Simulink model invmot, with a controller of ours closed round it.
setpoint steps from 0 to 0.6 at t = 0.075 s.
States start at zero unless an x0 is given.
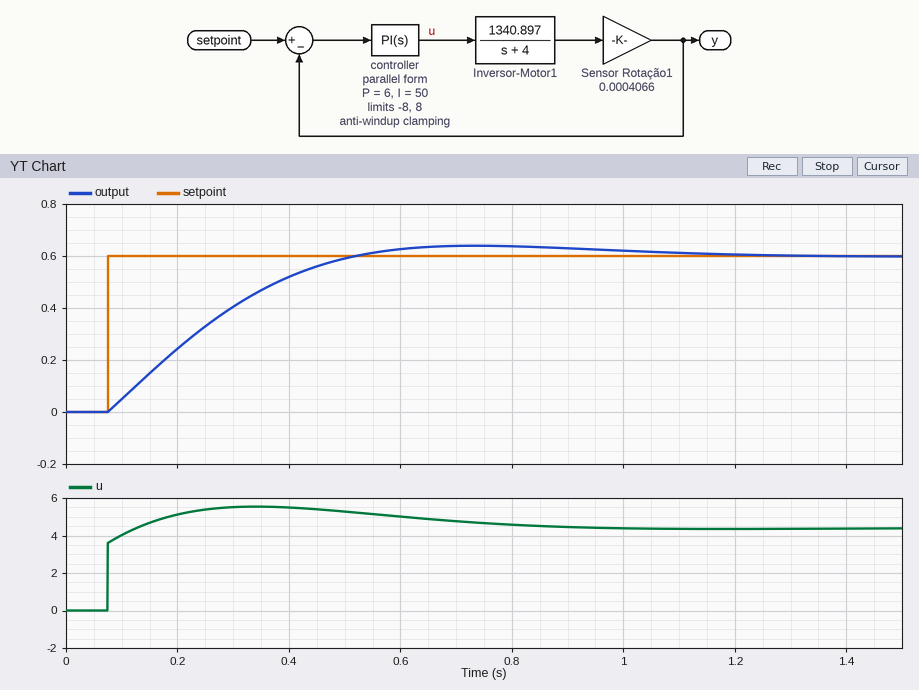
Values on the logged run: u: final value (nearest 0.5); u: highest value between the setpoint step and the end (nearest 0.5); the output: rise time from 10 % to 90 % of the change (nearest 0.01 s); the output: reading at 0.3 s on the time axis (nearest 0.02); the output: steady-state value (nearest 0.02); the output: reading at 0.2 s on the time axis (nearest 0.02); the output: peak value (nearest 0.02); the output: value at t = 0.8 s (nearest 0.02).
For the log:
4.5
5.5
0.32 s
0.40
0.60
0.24
0.64
0.64
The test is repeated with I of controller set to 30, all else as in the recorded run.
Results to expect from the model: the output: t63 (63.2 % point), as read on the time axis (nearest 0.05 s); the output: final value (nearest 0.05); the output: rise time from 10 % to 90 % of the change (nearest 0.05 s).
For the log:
0.35 s
0.60
0.50 s
